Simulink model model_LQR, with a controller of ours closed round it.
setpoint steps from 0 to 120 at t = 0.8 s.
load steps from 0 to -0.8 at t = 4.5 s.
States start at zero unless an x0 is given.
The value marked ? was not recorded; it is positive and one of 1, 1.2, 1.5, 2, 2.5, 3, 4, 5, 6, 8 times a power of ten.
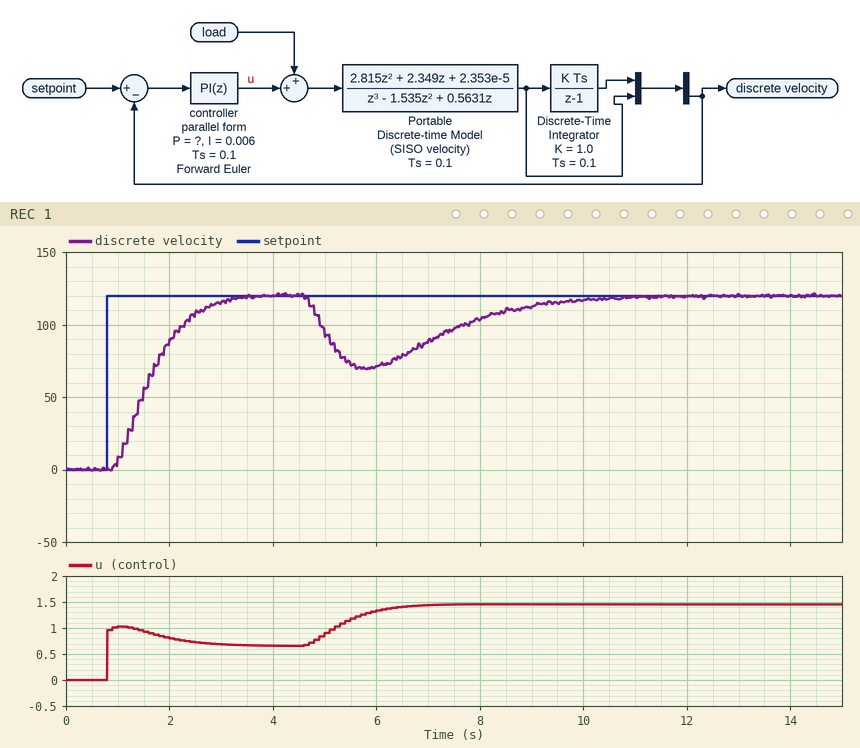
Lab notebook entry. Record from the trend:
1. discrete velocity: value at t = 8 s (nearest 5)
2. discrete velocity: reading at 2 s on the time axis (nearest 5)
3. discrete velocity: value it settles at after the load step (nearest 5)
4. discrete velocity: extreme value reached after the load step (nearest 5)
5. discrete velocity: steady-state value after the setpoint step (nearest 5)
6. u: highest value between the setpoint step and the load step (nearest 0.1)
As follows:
105
90
120
70
120
1.0
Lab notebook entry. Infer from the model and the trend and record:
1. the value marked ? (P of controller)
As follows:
0.008
